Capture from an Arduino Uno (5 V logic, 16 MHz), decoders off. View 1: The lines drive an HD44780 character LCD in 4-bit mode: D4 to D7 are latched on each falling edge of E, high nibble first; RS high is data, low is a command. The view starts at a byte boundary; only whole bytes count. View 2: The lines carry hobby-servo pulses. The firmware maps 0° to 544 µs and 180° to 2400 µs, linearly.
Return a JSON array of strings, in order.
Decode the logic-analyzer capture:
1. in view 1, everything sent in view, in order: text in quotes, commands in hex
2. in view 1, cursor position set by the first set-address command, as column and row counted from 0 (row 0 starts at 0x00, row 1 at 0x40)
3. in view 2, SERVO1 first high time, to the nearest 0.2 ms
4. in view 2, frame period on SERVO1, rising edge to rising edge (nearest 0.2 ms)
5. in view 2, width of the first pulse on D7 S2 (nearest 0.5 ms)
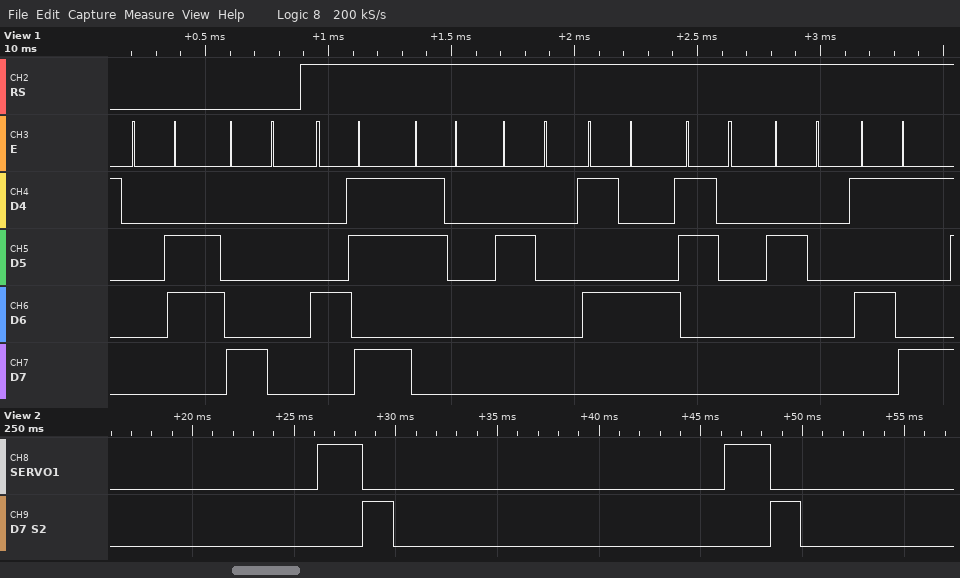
["0x06 0x80 \"K0 T0 Y\"", "column 0, row 0", "2.2 ms", "20.0 ms", "1.5 ms"]
